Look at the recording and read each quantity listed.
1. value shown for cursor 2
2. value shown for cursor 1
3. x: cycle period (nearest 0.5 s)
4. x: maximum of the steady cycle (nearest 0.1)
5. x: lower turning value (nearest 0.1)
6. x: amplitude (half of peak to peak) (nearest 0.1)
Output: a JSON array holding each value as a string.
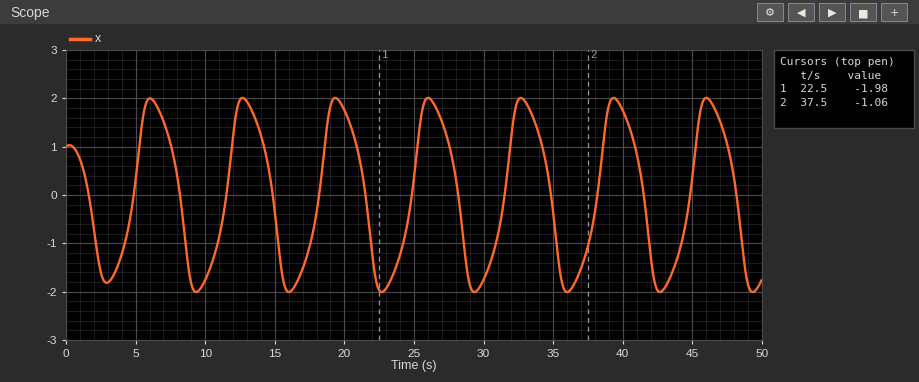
["-1.06", "-1.98", "6.5 s", "2.0", "-2.0", "2.0"]
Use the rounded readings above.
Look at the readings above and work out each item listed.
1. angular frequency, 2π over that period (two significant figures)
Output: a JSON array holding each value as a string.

["0.97 rad/s"]
